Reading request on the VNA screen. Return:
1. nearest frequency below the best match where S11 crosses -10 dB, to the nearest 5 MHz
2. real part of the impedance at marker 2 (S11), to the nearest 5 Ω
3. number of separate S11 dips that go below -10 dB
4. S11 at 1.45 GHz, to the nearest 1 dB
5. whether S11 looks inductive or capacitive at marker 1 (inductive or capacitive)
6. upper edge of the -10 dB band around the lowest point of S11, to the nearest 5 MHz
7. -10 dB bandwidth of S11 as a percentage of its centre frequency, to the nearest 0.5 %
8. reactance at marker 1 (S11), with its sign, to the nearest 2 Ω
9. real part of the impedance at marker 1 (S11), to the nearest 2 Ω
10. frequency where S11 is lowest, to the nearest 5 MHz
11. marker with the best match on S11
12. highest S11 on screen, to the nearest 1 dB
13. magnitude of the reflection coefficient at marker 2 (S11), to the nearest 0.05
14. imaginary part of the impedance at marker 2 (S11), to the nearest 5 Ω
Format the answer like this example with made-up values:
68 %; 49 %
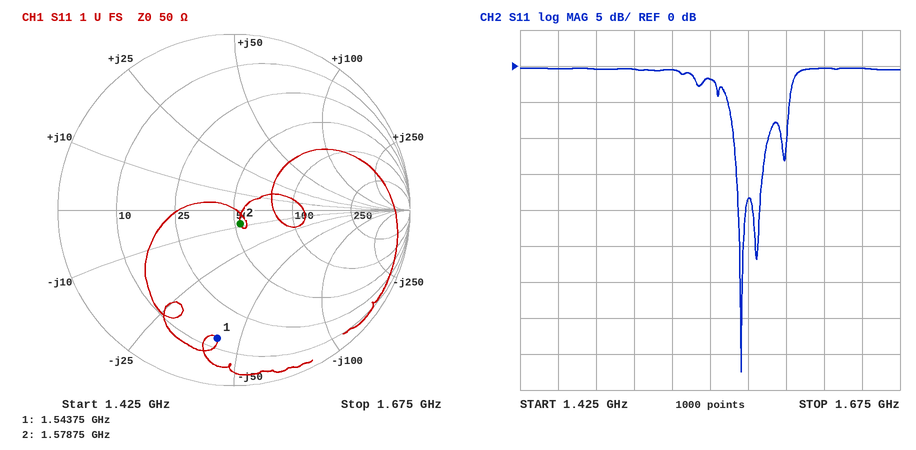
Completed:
1.565 GHz; 55 Ω; 3; 0 dB; capacitive; 1.590 GHz; 1.5 %; -42 Ω; 14 Ω; 1.570 GHz; marker 2; 0 dB; 0.10; -10 Ω
